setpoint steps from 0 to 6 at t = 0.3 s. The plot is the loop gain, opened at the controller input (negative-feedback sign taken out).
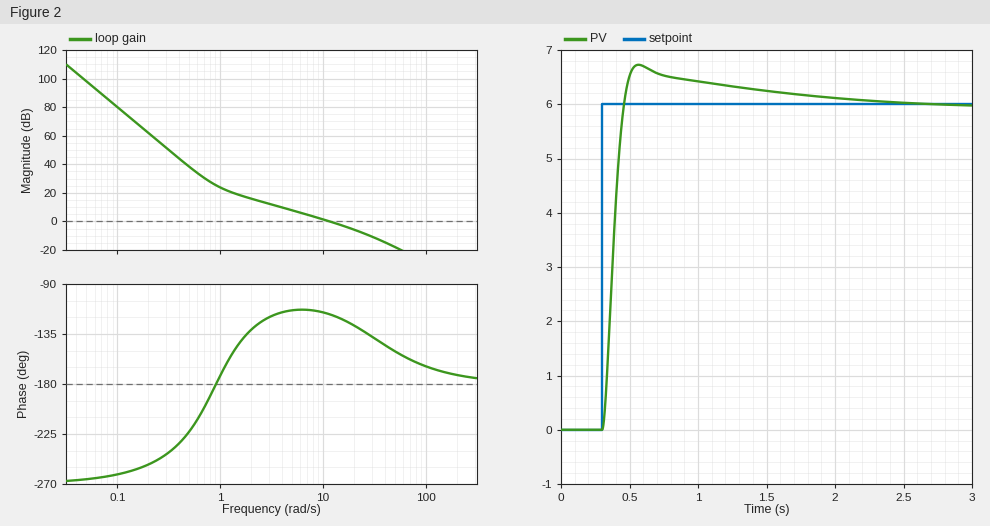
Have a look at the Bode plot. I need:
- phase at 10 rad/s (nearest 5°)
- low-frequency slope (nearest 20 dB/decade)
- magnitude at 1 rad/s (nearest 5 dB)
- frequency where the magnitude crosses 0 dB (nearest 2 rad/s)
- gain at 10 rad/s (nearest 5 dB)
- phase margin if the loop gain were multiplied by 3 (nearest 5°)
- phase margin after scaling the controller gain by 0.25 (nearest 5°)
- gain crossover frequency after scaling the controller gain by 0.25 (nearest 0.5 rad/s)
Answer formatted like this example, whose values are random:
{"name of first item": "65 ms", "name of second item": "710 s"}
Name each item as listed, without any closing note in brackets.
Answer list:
{"phase at 10 rad/s": "-115°", "low-frequency slope": "-60 dB/decade", "magnitude at 1 rad/s": "25 dB", "frequency where the magnitude crosses 0 dB": "12 rad/s", "gain at 10 rad/s": "0 dB", "phase margin if the loop gain were multiplied by 3": "45°", "phase margin after scaling the controller gain by 0.25": "60°", "gain crossover frequency after scaling the controller gain by 0.25": "3.0 rad/s"}
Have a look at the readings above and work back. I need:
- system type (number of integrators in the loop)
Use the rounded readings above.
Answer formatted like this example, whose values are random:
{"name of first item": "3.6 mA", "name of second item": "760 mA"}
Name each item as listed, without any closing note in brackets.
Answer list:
{"system type": "3"}
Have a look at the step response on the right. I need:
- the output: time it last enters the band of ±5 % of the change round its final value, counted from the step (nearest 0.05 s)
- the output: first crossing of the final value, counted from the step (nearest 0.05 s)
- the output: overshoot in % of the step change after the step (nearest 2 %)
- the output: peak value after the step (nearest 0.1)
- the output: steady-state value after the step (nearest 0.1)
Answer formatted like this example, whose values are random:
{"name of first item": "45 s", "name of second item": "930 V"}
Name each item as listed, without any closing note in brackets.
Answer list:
{"the output: time it last enters the band of ±5 % of the change round its final value, counted from the step": "1.05 s", "the output: first crossing of the final value, counted from the step": "0.15 s", "the output: overshoot in % of the step change after the step": "12 %", "the output: peak value after the step": "6.7", "the output: steady-state value after the step": "6.0"}
